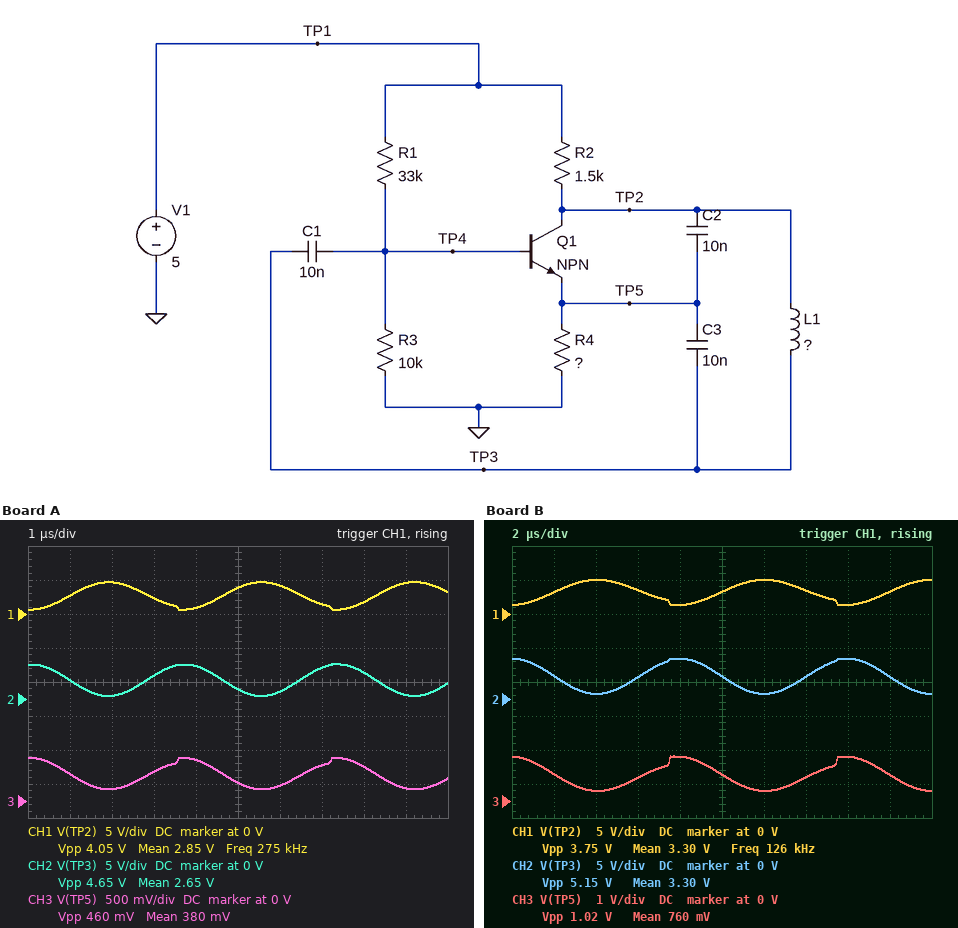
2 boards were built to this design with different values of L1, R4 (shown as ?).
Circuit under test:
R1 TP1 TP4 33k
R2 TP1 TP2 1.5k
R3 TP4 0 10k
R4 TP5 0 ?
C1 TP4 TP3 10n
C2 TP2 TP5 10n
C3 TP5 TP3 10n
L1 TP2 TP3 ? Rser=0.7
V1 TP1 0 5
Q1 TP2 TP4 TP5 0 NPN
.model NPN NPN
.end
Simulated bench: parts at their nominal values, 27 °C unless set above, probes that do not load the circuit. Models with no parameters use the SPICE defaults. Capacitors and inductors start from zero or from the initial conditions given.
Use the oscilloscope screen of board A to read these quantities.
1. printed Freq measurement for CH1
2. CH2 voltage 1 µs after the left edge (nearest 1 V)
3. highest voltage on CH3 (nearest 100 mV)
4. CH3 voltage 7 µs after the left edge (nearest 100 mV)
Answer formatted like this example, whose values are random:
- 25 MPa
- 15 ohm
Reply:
- 275 kHz
- 3 V
- 600 mV
- 500 mV
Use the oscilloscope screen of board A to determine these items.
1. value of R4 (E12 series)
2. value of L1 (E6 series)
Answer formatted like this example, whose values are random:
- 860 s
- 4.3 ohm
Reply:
- 220 Ω
- 68 µH
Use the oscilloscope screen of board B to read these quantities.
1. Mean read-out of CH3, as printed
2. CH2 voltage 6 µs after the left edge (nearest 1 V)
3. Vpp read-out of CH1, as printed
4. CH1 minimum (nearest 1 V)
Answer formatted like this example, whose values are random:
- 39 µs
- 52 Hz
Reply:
- 760 mV
- 3 V
- 3.75 V
- 1 V
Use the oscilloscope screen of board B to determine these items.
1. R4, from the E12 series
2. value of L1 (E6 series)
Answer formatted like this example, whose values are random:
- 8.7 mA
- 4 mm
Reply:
- 560 Ω
- 330 µH
